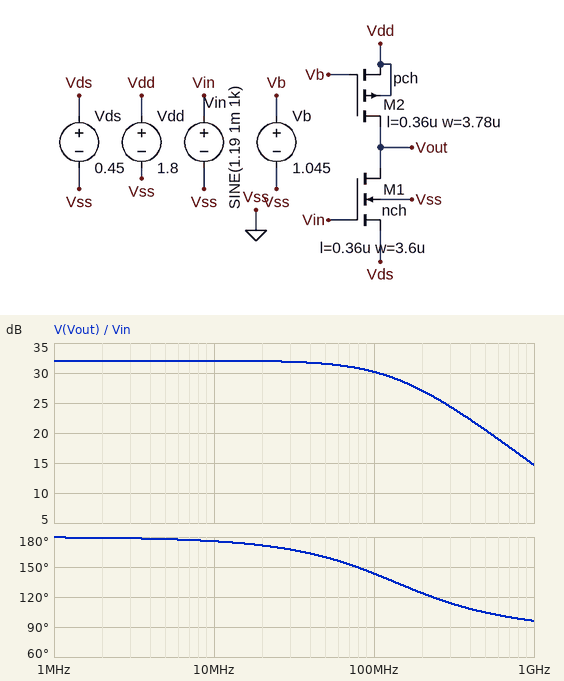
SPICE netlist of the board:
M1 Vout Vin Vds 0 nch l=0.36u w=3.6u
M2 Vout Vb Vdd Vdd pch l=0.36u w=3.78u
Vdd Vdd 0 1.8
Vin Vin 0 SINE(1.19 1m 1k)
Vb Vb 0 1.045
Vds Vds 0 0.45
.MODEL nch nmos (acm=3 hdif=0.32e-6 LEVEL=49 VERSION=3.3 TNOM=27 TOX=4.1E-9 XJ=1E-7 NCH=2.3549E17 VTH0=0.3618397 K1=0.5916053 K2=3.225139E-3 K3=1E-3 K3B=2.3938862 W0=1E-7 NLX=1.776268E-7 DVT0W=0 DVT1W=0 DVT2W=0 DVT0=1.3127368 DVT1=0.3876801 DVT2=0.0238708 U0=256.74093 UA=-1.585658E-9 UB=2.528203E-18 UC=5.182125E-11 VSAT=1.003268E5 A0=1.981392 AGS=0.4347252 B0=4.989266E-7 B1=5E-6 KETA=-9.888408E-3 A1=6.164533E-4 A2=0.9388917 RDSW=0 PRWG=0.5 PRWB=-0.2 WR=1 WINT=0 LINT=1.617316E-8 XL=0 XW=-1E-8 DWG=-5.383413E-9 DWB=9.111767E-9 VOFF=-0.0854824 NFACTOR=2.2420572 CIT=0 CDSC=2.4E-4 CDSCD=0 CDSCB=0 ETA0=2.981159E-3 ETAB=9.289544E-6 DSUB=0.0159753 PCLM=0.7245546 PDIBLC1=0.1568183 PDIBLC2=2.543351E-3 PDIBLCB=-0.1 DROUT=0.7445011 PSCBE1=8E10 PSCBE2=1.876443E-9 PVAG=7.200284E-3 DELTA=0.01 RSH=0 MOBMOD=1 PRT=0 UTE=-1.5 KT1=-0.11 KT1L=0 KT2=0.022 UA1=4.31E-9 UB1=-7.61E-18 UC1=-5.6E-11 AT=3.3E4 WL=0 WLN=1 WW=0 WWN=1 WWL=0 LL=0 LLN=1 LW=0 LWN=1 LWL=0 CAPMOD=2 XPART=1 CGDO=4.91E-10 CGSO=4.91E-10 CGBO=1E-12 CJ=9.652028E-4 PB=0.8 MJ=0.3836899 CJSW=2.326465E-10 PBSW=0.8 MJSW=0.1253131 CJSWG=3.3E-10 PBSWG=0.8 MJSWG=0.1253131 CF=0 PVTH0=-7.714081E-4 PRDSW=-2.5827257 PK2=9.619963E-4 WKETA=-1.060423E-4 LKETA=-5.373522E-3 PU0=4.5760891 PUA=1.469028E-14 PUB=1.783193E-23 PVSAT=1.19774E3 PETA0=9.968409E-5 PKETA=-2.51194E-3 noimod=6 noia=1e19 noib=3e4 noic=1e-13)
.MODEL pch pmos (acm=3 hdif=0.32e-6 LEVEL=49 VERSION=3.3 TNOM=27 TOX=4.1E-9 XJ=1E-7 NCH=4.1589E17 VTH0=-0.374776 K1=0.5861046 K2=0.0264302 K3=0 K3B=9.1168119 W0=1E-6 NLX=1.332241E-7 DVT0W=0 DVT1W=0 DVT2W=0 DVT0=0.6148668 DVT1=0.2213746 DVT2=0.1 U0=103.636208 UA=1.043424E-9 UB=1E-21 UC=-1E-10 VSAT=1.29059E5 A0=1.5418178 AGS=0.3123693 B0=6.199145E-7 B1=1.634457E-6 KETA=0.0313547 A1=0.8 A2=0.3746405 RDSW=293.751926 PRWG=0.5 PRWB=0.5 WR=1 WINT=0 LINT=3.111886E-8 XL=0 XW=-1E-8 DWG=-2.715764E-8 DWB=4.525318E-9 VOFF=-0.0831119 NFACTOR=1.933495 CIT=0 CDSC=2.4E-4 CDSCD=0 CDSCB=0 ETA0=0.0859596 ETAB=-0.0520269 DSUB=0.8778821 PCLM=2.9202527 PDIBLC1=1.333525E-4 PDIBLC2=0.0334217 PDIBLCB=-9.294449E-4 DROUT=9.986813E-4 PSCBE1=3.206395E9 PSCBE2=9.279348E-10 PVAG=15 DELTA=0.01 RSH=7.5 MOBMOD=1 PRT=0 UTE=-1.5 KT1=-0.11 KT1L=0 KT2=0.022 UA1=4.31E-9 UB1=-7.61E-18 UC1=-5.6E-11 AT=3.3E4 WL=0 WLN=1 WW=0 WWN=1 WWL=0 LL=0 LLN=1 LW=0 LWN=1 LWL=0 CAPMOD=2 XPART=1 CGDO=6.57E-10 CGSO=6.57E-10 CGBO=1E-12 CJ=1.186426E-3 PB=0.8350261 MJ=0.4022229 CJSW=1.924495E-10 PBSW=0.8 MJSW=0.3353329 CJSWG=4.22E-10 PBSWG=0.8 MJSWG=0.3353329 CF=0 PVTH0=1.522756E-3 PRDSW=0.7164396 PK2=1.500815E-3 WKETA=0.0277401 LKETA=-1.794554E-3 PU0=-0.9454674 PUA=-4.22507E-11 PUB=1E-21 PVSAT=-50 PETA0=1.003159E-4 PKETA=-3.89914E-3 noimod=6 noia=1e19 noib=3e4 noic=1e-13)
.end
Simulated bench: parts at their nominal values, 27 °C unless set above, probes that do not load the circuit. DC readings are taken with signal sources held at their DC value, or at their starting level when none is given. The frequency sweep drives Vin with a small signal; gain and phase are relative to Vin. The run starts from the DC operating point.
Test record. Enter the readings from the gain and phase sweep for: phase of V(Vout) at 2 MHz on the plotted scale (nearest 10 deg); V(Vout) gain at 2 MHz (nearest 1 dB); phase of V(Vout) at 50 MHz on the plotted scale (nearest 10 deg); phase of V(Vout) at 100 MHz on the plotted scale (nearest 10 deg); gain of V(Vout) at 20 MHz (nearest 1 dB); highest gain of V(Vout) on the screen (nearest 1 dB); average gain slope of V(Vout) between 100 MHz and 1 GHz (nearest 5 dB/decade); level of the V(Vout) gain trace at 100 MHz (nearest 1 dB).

180 deg
32 dB
160 deg
140 deg
32 dB
32 dB
-15 dB/decade
30 dB
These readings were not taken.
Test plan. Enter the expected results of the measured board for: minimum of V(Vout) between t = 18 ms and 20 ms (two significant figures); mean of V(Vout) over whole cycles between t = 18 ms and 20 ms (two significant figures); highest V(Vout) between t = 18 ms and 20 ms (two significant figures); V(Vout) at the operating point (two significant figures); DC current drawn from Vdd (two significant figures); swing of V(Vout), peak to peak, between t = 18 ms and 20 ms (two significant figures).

1.0 V
1.1 V
1.1 V
1.1 V
35 µA
80 mV
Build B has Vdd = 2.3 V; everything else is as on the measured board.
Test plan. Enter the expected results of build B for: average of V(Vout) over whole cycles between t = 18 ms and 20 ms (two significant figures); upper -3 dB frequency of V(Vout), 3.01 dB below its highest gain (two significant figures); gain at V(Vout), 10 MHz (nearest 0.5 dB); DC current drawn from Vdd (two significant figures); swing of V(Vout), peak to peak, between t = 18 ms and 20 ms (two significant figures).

2.2 V
3.2 GHz
-1.0 dB
41 µA
1.8 mV
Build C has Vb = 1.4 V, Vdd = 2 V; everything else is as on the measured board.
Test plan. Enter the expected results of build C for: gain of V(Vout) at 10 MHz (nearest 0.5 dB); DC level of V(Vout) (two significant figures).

-11.5 dB
480 mV
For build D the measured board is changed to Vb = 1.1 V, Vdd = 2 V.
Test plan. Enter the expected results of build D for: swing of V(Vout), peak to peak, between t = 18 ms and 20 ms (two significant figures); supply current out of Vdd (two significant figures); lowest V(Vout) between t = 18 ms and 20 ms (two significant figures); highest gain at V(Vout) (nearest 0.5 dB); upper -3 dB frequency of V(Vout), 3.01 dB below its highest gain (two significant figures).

4.1 mV
39 µA
1.9 V
6.0 dB
1.7 GHz
